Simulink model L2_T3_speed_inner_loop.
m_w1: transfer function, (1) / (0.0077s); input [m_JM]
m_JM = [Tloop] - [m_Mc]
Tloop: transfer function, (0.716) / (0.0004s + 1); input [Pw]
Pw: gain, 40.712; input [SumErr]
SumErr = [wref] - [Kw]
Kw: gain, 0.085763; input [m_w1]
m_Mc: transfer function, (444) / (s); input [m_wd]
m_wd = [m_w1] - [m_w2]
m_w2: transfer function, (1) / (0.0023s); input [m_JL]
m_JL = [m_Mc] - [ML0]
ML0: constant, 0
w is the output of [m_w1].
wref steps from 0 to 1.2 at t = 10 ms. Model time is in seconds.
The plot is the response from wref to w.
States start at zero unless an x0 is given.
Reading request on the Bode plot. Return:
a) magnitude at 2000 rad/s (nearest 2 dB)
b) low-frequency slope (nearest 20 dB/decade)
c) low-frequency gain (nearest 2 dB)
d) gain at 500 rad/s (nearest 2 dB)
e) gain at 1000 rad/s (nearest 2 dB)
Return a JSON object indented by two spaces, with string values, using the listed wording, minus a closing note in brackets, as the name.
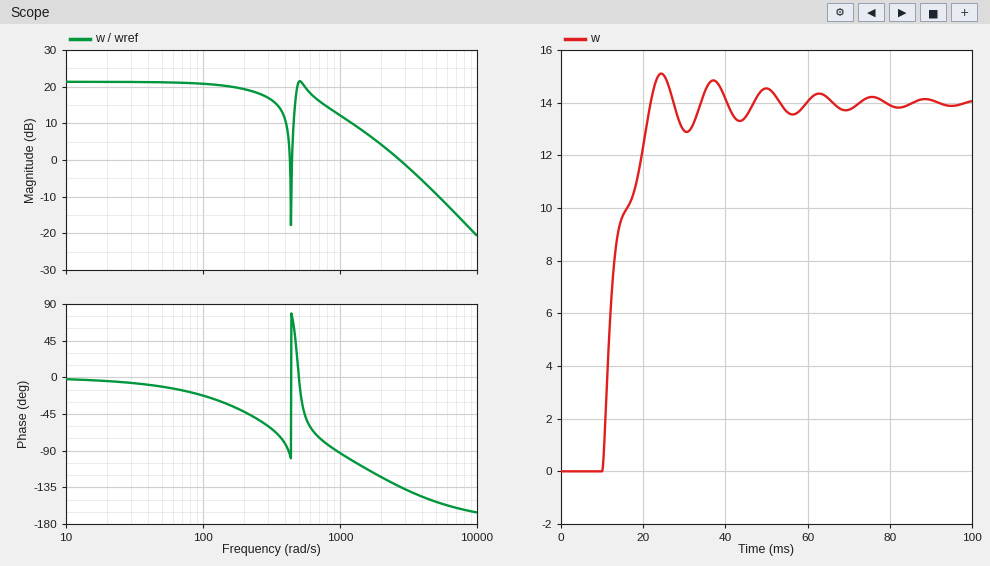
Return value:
{
  "magnitude at 2000 rad/s": "4 dB",
  "low-frequency slope": "0 dB/decade",
  "low-frequency gain": "22 dB",
  "gain at 500 rad/s": "22 dB",
  "gain at 1000 rad/s": "12 dB"
}
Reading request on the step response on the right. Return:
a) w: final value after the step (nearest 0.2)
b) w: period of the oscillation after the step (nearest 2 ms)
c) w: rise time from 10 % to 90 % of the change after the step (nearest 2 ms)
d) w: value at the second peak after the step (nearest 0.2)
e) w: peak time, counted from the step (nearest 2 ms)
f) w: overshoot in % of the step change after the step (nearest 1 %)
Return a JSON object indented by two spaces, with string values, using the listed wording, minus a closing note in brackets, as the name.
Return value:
{
  "w: final value after the step": "14.0",
  "w: period of the oscillation after the step": "12 ms",
  "w: rise time from 10 % to 90 % of the change after the step": "10 ms",
  "w: value at the second peak after the step": "14.8",
  "w: peak time, counted from the step": "14 ms",
  "w: overshoot in % of the step change after the step": "8 %"
}
